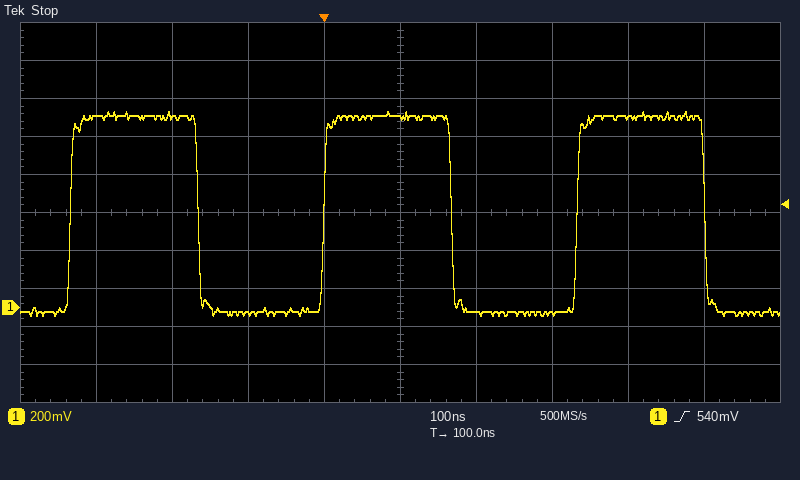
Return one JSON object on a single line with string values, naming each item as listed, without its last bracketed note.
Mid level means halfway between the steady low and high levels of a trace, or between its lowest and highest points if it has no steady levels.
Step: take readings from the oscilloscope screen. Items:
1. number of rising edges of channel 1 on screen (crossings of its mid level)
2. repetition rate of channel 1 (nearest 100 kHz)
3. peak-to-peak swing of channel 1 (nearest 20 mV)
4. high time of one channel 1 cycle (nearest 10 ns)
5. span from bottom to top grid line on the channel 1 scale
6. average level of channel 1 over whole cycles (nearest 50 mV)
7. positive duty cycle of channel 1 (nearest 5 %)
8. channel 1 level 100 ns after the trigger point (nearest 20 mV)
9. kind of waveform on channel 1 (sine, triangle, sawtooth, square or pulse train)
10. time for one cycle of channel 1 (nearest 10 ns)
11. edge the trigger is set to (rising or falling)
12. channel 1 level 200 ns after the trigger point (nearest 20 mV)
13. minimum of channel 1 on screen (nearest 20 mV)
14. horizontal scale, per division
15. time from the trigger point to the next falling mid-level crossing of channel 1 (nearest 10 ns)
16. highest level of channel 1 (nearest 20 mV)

{"number of rising edges of channel 1 on screen": "3", "repetition rate of channel 1": "3.0 MHz", "peak-to-peak swing of channel 1": "1.08 V", "high time of one channel 1 cycle": "170 ns", "span from bottom to top grid line on the channel 1 scale": "2 V", "average level of channel 1 over whole cycles": "500 mV", "positive duty cycle of channel 1": "50 %", "channel 1 level 100 ns after the trigger point": "1.00 V", "kind of waveform on channel 1": "square", "time for one cycle of channel 1": "330 ns", "edge the trigger is set to": "rising", "channel 1 level 200 ns after the trigger point": "-20 mV", "minimum of channel 1 on screen": "-40 mV", "horizontal scale, per division": "100 ns", "time from the trigger point to the next falling mid-level crossing of channel 1": "170 ns", "highest level of channel 1": "1.04 V"}
